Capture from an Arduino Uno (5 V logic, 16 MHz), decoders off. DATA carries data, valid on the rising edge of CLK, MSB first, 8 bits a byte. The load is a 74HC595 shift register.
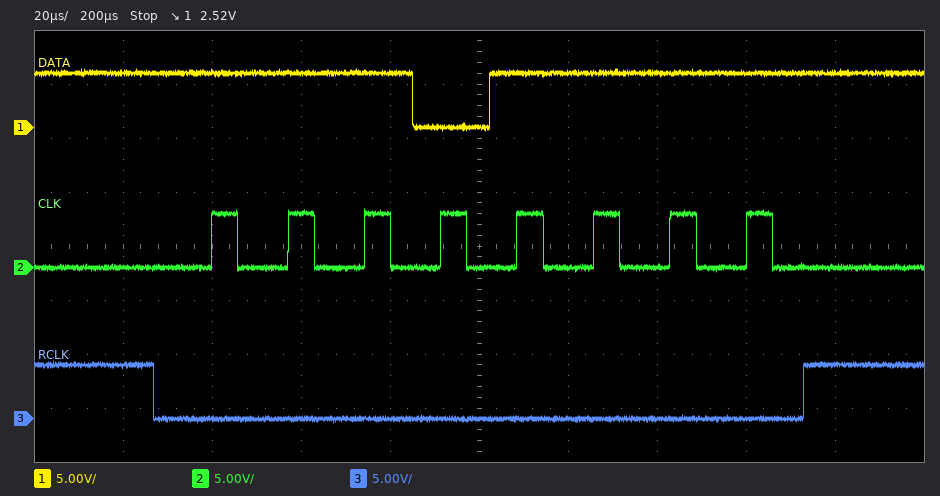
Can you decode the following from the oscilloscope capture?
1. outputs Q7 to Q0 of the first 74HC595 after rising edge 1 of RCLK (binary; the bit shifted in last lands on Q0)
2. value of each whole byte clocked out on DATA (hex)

11101111
EF
